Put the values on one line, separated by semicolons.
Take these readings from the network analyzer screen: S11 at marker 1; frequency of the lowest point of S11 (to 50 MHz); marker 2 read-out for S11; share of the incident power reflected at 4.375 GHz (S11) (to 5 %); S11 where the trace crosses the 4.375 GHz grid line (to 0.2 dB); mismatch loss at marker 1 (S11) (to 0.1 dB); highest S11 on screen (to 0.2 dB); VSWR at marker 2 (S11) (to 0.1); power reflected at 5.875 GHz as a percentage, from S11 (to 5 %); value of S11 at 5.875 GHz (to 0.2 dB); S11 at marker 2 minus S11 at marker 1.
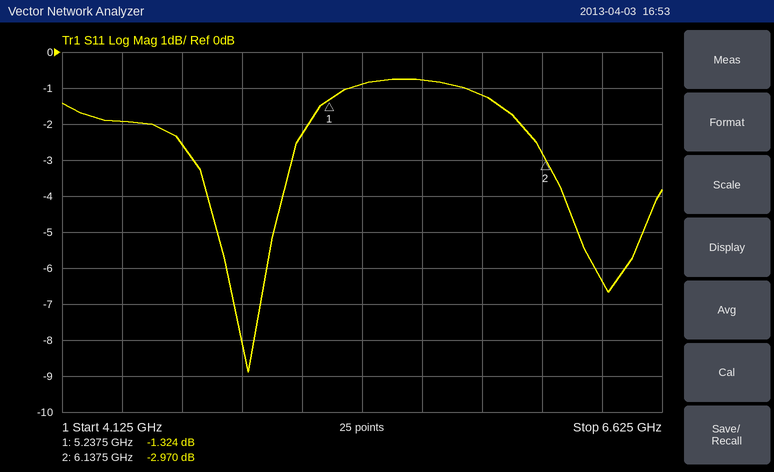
-1.324 dB; 4.90 GHz; -2.970 dB; 65 %; -2.0 dB; 5.8 dB; -0.8 dB; 5.9; 75 %; -1.2 dB; -1.646 dB
